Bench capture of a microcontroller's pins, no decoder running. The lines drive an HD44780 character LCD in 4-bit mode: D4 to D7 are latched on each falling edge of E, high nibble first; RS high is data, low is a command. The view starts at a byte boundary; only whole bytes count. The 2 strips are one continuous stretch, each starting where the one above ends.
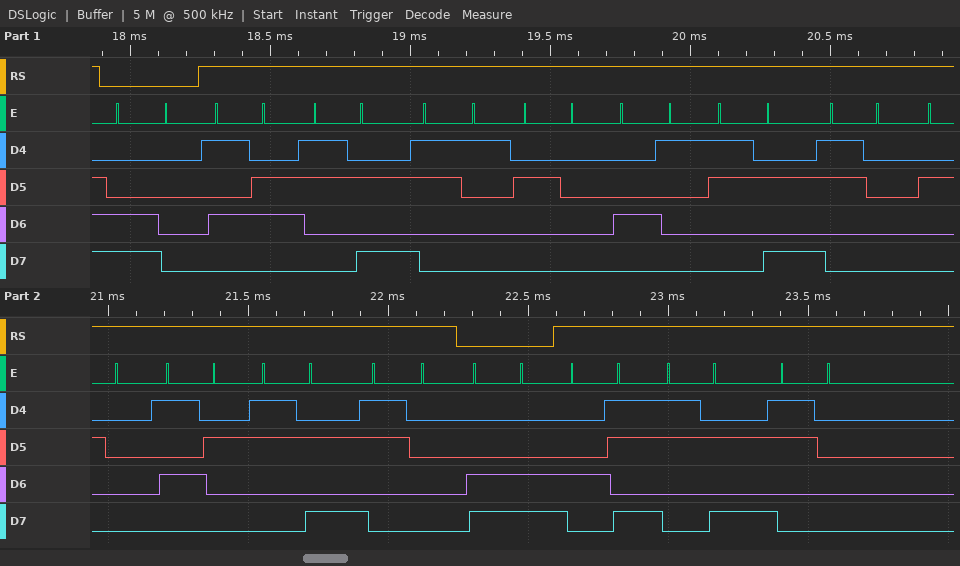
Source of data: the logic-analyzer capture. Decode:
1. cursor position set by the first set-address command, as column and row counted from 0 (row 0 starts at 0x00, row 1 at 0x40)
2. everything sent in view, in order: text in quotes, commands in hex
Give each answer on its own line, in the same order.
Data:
column 0, row 1
0xC0 "V:1 A:0 R:0" 0xCC "K:0"
